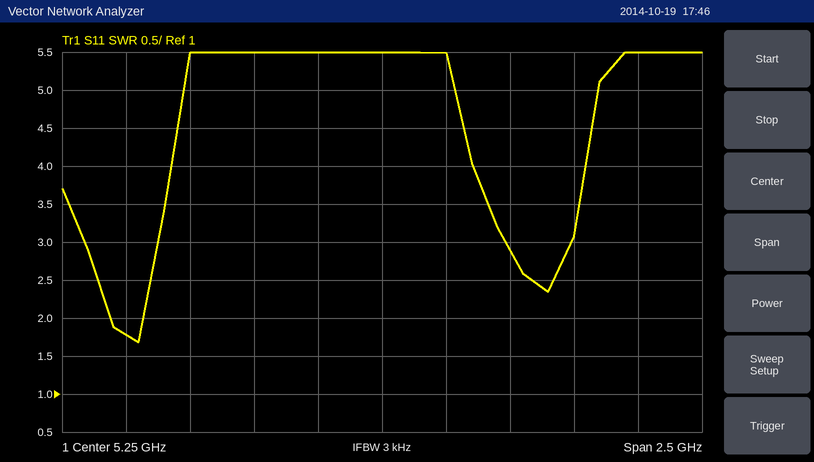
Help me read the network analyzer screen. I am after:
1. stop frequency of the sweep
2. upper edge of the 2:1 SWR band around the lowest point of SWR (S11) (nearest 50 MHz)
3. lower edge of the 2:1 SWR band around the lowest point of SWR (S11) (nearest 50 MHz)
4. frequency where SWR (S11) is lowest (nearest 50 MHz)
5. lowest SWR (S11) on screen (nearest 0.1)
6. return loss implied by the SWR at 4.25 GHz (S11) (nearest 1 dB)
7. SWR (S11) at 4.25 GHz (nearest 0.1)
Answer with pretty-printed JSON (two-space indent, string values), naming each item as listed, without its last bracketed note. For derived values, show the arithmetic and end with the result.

{
  "stop frequency of the sweep": "6.5 GHz",
  "upper edge of the 2:1 SWR band around the lowest point of SWR (S11)": "4.30 GHz",
  "lower edge of the 2:1 SWR band around the lowest point of SWR (S11)": "4.20 GHz",
  "frequency where SWR (S11) is lowest": "4.30 GHz",
  "lowest SWR (S11) on screen": "1.7",
  "return loss implied by the SWR at 4.25 GHz (S11)": "−20 log10((1.8 − 1)/(1.8 + 1)) ≈ 11 dB",
  "SWR (S11) at 4.25 GHz": "1.8"
}
